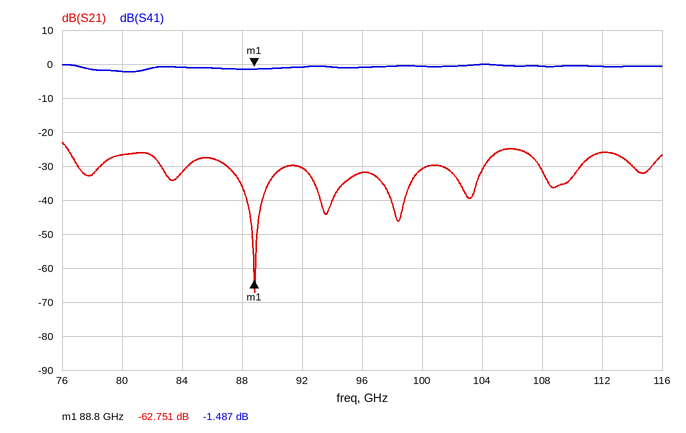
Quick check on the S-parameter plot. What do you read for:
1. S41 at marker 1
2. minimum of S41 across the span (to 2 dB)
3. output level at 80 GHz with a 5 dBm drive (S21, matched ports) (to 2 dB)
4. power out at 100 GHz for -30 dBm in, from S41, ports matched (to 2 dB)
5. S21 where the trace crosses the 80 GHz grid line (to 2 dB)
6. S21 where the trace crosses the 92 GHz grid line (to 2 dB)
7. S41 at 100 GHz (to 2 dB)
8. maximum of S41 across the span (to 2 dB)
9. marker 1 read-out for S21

-1.487 dB
-2 dB
-22 dBm
-30 dBm
-26 dB
-30 dB
0 dB
0 dB
-62.751 dB
